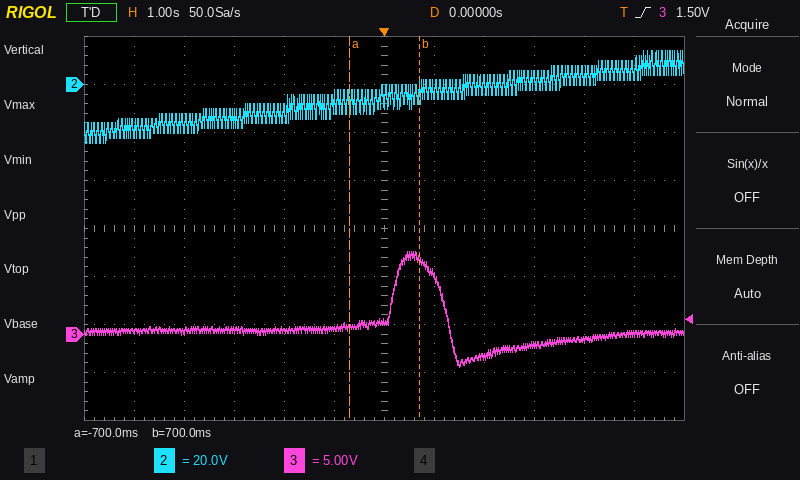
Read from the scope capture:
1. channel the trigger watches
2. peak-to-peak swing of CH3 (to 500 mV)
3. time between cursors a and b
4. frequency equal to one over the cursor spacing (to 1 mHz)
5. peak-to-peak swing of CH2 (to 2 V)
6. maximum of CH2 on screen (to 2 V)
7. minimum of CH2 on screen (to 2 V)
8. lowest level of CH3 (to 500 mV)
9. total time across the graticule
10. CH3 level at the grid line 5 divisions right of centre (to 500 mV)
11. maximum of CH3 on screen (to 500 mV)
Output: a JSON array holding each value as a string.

["CH3", "12.0 V", "1.4 s", "714 mHz", "38 V", "14 V", "-24 V", "-3.5 V", "12 s", "0.0 V", "8.5 V"]
